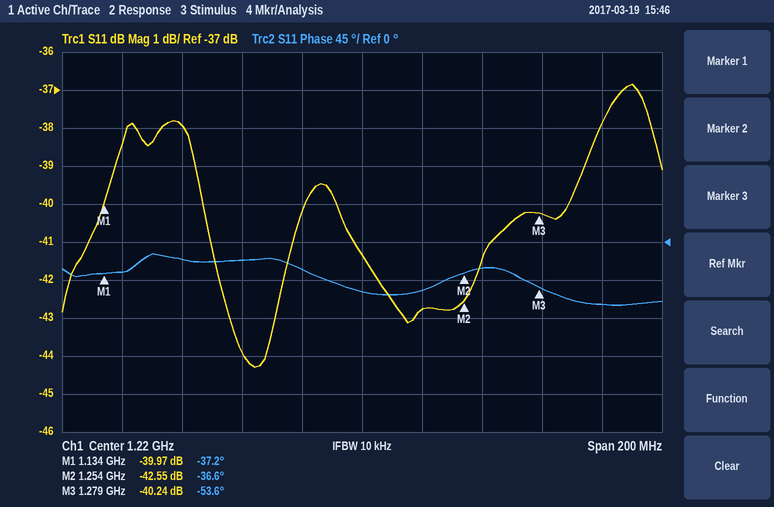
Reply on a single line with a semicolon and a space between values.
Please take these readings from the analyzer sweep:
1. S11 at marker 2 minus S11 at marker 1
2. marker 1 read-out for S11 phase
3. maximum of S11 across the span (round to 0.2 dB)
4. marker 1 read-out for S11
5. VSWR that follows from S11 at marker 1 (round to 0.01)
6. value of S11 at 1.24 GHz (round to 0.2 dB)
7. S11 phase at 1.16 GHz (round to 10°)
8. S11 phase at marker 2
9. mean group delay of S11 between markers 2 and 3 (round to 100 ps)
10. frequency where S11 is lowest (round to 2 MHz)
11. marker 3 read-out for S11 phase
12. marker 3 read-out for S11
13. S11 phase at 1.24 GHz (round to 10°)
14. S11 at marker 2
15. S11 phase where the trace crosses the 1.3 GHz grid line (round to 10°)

-2.58 dB; -37.2°; -36.8 dB; -39.97 dB; 1.02; -42.8 dB; -20°; -36.6°; 1.9 ns; 1.184 GHz; -53.6°; -40.24 dB; -60°; -42.55 dB; -70°
